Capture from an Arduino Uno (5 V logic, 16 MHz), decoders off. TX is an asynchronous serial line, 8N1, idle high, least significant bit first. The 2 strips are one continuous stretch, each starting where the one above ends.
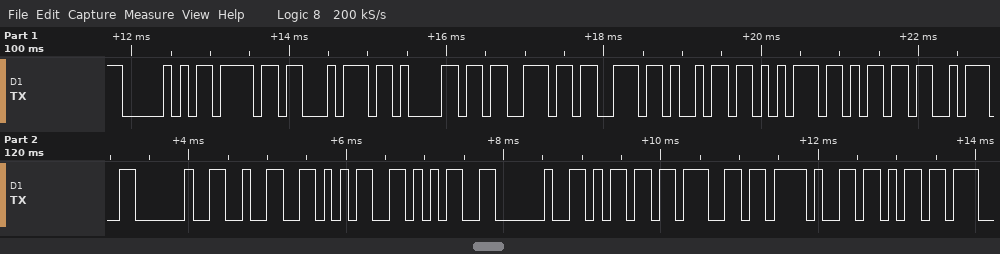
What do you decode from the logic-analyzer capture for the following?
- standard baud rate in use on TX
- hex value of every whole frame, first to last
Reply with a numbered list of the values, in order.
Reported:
1. 9600 baud
2. 50 6F 74 61 73 73 69 75 6D 3A 20 32 35 35 20 6D 67 2F 6B
